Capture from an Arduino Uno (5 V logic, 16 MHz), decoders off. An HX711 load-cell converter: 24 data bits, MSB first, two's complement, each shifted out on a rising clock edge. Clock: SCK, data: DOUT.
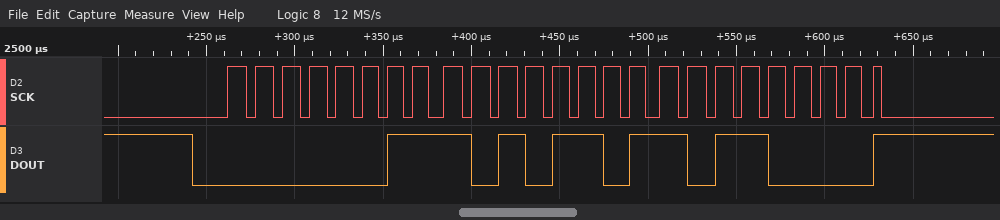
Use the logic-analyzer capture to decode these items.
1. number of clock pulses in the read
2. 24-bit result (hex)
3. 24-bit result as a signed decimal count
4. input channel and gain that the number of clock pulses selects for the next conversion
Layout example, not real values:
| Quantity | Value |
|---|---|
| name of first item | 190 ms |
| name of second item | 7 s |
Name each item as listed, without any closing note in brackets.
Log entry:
| Quantity | Value |
|---|---|
| number of clock pulses in the read | 25 |
| 24-bit result | 0x03ADB0 |
| 24-bit result as a signed decimal count | 241072 |
| input channel and gain that the number of clock pulses selects for the next conversion | channel A, gain 128 |
